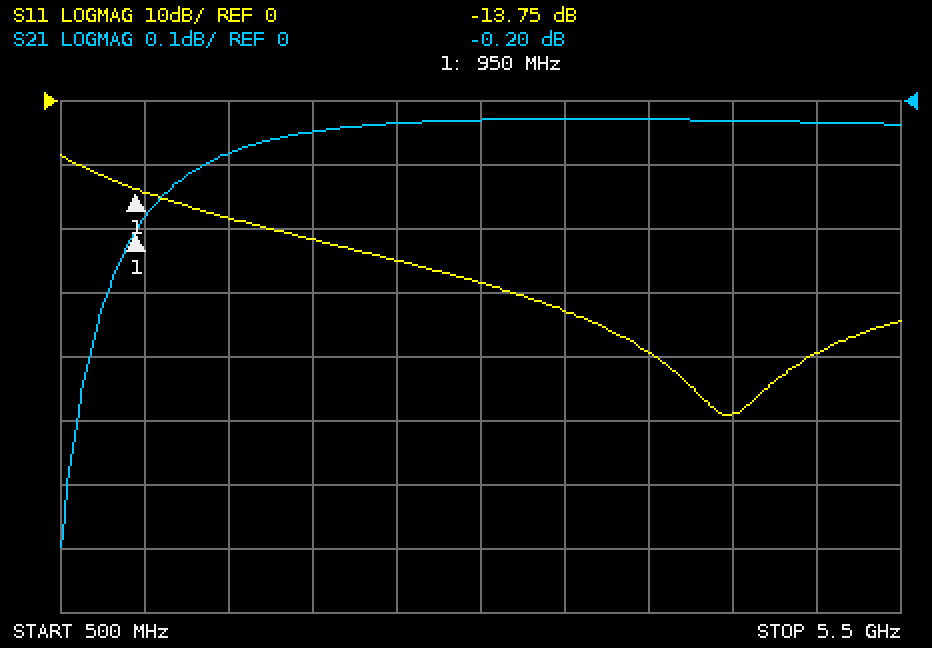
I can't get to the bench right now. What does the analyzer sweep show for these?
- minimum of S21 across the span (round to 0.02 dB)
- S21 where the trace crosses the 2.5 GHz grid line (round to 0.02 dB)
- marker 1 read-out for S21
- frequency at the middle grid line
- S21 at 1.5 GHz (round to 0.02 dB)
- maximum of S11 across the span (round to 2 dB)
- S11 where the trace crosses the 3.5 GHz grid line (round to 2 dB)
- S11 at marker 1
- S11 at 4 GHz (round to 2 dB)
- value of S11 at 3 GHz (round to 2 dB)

-0.70 dB
-0.04 dB
-0.20 dB
3 GHz
-0.08 dB
-8 dB
-32 dB
-13.75 dB
-40 dB
-28 dB
